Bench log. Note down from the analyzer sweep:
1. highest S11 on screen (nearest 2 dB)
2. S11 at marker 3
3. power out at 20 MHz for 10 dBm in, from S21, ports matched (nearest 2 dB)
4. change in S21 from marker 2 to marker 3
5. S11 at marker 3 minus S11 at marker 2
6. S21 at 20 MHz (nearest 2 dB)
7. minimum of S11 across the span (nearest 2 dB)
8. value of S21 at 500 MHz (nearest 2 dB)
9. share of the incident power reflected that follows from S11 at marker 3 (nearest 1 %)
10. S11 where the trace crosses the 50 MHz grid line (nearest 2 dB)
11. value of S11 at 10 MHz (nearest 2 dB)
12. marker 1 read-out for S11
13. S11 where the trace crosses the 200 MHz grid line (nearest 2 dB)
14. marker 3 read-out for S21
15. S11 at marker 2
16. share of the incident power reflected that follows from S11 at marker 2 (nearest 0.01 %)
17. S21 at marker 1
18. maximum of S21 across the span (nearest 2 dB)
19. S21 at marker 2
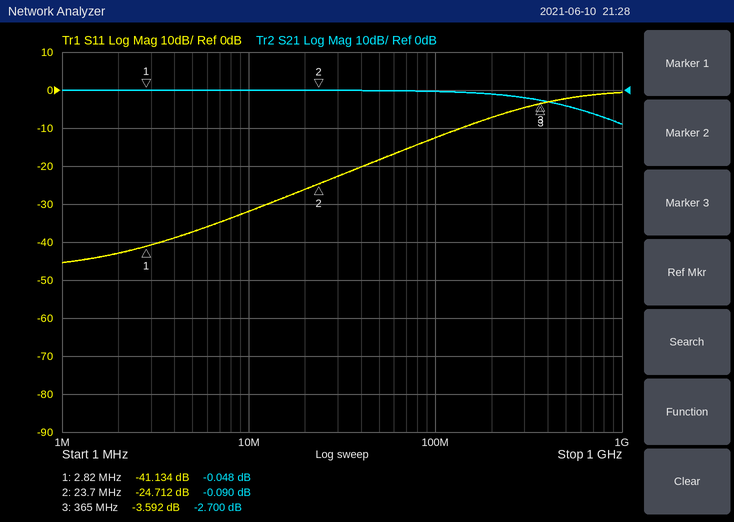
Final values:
0 dB
-3.592 dB
10 dBm
-2.610 dB
21.120 dB
0 dB
-46 dB
-4 dB
44 %
-18 dB
-32 dB
-41.134 dB
-8 dB
-2.700 dB
-24.712 dB
0.34 %
-0.048 dB
0 dB
-0.090 dB
